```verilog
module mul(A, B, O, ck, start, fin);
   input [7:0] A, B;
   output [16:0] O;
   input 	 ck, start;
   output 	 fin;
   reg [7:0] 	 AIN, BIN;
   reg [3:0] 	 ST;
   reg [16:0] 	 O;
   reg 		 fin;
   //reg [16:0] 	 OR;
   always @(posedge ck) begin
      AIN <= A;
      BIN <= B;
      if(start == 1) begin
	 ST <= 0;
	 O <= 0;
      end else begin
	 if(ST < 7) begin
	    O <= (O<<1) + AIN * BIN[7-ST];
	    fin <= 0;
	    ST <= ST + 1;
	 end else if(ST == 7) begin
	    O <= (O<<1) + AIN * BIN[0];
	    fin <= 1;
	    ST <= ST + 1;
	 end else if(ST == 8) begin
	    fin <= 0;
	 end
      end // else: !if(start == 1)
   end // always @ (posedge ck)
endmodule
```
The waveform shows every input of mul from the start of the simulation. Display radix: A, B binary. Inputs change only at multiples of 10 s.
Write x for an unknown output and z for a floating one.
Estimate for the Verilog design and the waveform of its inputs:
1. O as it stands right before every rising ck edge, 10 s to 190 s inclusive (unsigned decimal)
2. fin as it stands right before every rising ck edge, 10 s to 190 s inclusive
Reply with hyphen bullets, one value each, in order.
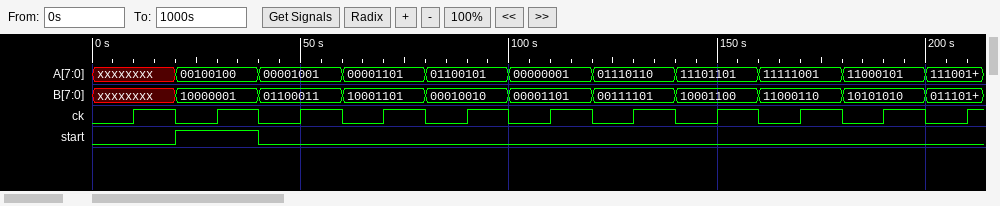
- x, x, 0, 36, 81, 162, 425, 851, 1820, 3640
- x x x 0 0 0 0 0 0 0
